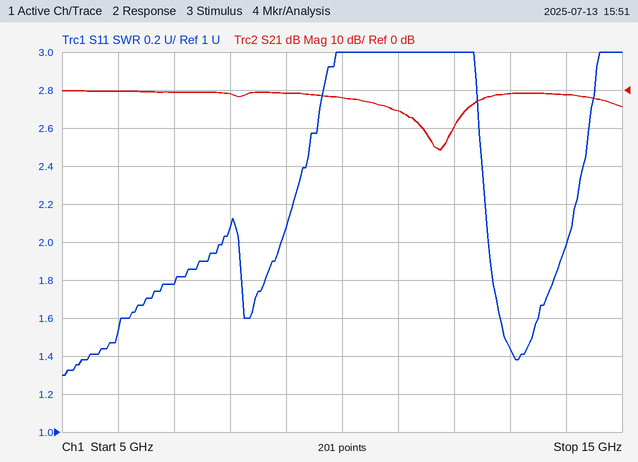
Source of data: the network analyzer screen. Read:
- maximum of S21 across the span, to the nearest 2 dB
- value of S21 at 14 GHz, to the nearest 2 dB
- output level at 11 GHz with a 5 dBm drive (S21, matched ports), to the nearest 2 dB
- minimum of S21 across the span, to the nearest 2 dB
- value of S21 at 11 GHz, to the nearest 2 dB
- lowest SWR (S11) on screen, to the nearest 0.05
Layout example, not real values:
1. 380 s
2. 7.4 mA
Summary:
1. 0 dB
2. -2 dB
3. 0 dBm
4. -16 dB
5. -6 dB
6. 1.30
